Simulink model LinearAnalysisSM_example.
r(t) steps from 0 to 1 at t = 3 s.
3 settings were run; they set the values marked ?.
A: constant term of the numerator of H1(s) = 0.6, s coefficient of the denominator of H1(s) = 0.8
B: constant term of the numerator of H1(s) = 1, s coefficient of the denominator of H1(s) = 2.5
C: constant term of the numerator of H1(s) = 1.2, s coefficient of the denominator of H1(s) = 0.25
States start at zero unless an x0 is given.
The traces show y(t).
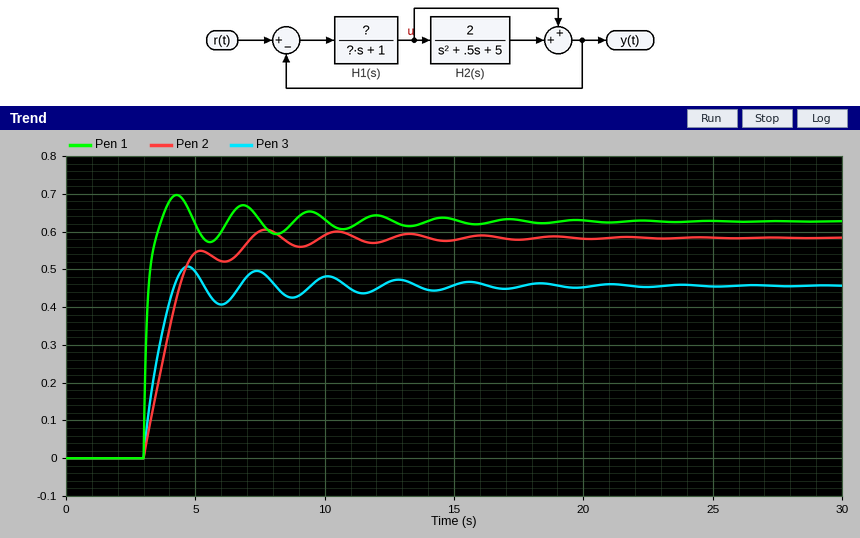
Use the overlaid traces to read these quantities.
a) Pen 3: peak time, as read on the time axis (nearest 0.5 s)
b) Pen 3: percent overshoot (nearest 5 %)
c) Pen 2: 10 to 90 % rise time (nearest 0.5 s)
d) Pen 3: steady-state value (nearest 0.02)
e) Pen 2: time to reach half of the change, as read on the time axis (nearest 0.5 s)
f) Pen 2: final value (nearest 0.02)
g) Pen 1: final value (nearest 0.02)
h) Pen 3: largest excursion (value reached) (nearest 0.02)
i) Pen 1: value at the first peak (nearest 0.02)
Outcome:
4.5 s
10 %
1.5 s
0.46
4.0 s
0.58
0.62
0.50
0.70
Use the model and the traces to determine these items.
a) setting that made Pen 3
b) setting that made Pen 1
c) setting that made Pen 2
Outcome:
A
C
B
